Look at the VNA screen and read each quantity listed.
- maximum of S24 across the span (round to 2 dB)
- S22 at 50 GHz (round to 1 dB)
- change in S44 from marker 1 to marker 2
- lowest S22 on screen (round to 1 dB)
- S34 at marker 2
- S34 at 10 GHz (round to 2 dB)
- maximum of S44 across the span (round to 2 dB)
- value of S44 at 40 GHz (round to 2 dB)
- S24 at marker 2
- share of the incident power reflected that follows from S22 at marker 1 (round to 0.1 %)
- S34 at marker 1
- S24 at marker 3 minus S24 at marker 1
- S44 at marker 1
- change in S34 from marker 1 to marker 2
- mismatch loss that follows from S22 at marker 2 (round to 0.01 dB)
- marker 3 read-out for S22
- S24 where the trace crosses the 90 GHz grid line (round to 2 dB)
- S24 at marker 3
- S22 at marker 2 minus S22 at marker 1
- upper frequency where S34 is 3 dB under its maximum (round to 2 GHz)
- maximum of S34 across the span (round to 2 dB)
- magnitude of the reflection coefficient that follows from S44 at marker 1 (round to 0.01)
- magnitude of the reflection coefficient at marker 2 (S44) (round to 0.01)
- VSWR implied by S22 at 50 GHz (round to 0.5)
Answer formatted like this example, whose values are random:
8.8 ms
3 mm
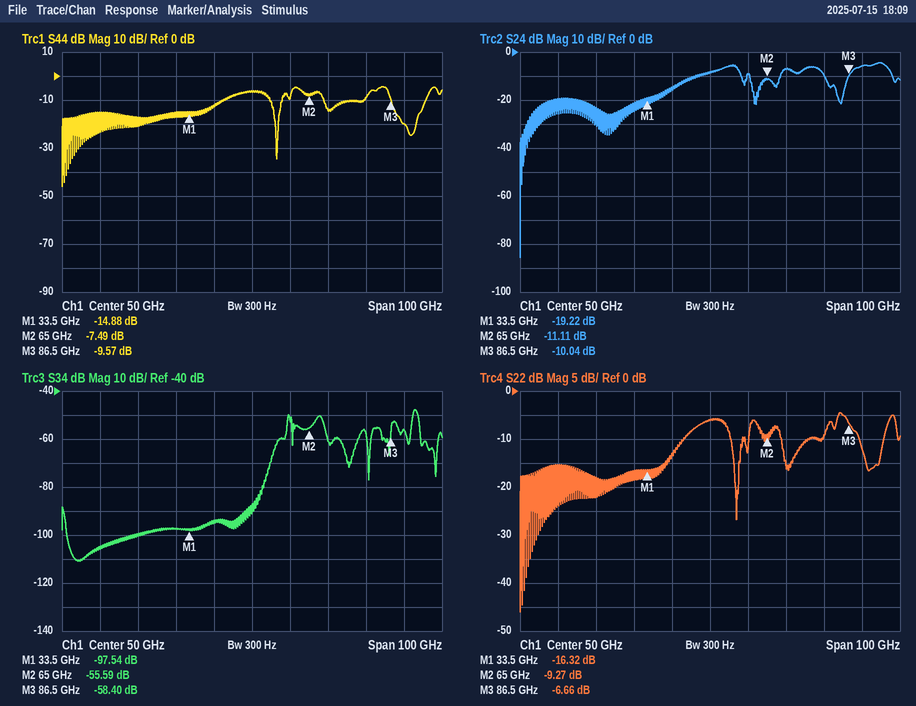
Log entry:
-4 dB
-6 dB
7.39 dB
-46 dB
-55.59 dB
-106 dB
-4 dB
-12 dB
-11.11 dB
2.3 %
-97.54 dB
9.18 dB
-14.88 dB
41.95 dB
0.55 dB
-6.66 dB
-6 dB
-10.04 dB
7.05 dB
94 GHz
-48 dB
0.18
0.42
3.0
